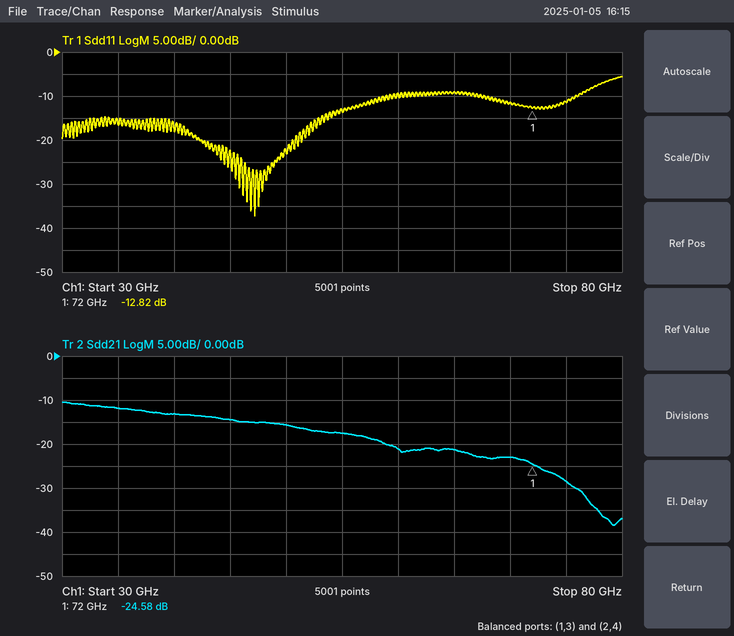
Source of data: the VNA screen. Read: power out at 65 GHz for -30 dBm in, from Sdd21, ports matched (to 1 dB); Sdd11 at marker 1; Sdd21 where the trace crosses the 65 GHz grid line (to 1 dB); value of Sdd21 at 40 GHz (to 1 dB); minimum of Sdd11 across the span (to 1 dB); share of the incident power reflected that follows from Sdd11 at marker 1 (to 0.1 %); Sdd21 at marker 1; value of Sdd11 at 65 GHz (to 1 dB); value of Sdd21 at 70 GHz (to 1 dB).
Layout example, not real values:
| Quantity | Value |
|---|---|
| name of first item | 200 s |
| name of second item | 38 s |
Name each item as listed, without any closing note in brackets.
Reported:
| Quantity | Value |
|---|---|
| power out at 65 GHz for -30 dBm in, from Sdd21, ports matched | -51 dBm |
| Sdd11 at marker 1 | -12.82 dB |
| Sdd21 where the trace crosses the 65 GHz grid line | -21 dB |
| value of Sdd21 at 40 GHz | -13 dB |
| minimum of Sdd11 across the span | -37 dB |
| share of the incident power reflected that follows from Sdd11 at marker 1 | 5.2 % |
| Sdd21 at marker 1 | -24.58 dB |
| value of Sdd11 at 65 GHz | -9 dB |
| value of Sdd21 at 70 GHz | -23 dB |
